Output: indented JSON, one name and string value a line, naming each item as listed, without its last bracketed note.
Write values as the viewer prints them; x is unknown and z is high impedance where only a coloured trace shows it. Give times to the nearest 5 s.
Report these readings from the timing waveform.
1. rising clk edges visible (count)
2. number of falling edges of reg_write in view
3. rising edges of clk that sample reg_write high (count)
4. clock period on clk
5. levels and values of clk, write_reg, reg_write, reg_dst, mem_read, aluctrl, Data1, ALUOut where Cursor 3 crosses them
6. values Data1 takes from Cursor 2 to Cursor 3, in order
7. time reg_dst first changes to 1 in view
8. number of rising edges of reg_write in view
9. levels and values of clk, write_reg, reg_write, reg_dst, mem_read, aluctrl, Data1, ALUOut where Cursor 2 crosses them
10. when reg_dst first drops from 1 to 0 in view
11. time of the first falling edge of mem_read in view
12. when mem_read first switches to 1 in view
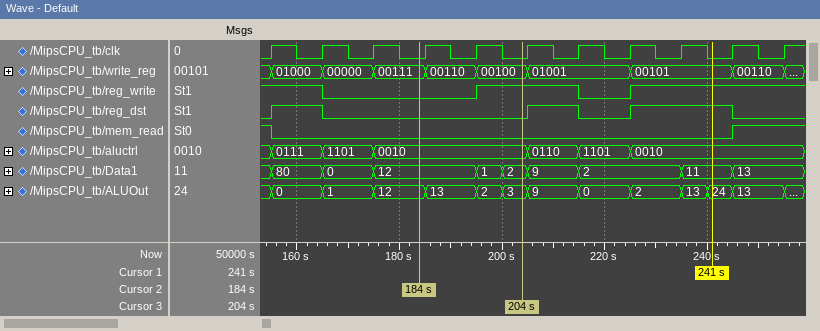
{
  "rising clk edges visible": "11",
  "number of falling edges of reg_write in view": "2",
  "rising edges of clk that sample reg_write high": "7",
  "clock period on clk": "10 s",
  "levels and values of clk, write_reg, reg_write, reg_dst, mem_read, aluctrl, Data1, ALUOut where Cursor 3 crosses them": "clk=0, write_reg=00100, reg_write=1, reg_dst=0, mem_read=0, aluctrl=0010, Data1=2, ALUOut=3",
  "values Data1 takes from Cursor 2 to Cursor 3, in order": "12, 1, 2",
  "time reg_dst first changes to 1 in view": "155 s",
  "number of rising edges of reg_write in view": "2",
  "levels and values of clk, write_reg, reg_write, reg_dst, mem_read, aluctrl, Data1, ALUOut where Cursor 2 crosses them": "clk=0, write_reg=00111, reg_write=0, reg_dst=0, mem_read=0, aluctrl=0010, Data1=12, ALUOut=12",
  "when reg_dst first drops from 1 to 0 in view": "165 s",
  "time of the first falling edge of mem_read in view": "155 s",
  "when mem_read first switches to 1 in view": "245 s"
}
